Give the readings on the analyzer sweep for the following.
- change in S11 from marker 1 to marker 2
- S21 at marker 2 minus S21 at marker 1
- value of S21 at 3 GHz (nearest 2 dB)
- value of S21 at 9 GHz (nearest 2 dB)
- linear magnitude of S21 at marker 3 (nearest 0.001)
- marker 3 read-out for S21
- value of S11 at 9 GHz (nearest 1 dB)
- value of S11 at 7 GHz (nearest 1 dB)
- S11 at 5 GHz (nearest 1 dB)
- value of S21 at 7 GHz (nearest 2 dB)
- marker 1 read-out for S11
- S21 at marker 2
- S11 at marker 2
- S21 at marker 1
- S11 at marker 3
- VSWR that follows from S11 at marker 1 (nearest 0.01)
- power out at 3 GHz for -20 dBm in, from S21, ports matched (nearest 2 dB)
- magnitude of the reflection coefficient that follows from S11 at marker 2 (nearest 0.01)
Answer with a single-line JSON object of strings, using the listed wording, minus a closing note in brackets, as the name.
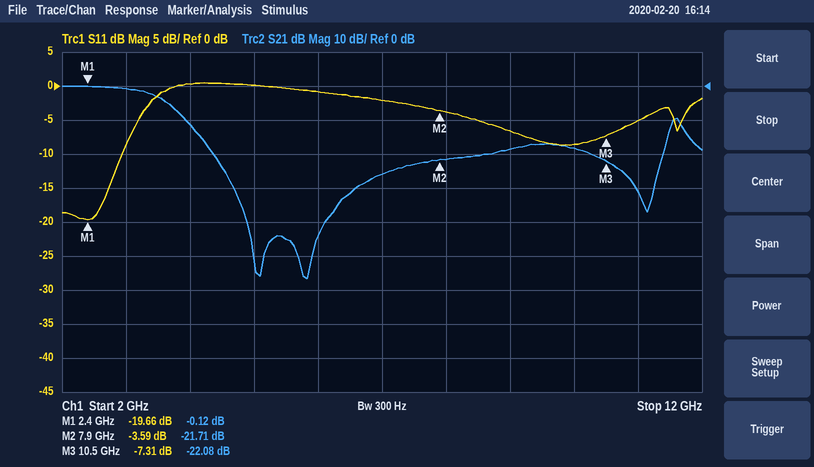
{"change in S11 from marker 1 to marker 2": "16.07 dB", "S21 at marker 2 minus S21 at marker 1": "-21.59 dB", "value of S21 at 3 GHz": "0 dB", "value of S21 at 9 GHz": "-18 dB", "linear magnitude of S21 at marker 3": "0.079", "marker 3 read-out for S21": "-22.08 dB", "value of S11 at 9 GHz": "-7 dB", "value of S11 at 7 GHz": "-2 dB", "S11 at 5 GHz": "0 dB", "value of S21 at 7 GHz": "-26 dB", "marker 1 read-out for S11": "-19.66 dB", "S21 at marker 2": "-21.71 dB", "S11 at marker 2": "-3.59 dB", "S21 at marker 1": "-0.12 dB", "S11 at marker 3": "-7.31 dB", "VSWR that follows from S11 at marker 1": "1.23", "power out at 3 GHz for -20 dBm in, from S21, ports matched": "-20 dBm", "magnitude of the reflection coefficient that follows from S11 at marker 2": "0.66"}
